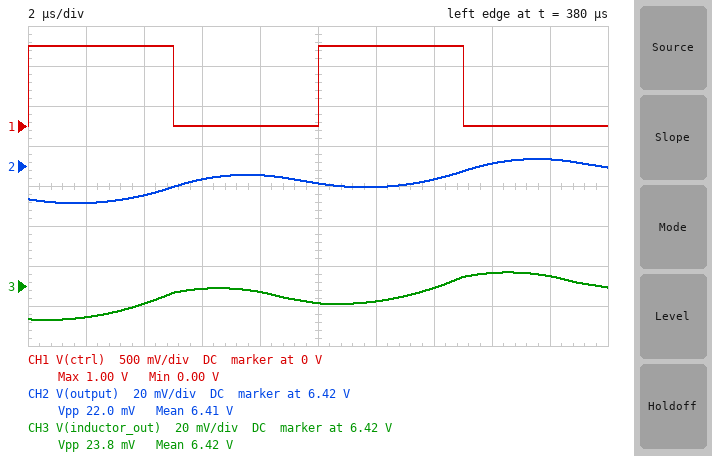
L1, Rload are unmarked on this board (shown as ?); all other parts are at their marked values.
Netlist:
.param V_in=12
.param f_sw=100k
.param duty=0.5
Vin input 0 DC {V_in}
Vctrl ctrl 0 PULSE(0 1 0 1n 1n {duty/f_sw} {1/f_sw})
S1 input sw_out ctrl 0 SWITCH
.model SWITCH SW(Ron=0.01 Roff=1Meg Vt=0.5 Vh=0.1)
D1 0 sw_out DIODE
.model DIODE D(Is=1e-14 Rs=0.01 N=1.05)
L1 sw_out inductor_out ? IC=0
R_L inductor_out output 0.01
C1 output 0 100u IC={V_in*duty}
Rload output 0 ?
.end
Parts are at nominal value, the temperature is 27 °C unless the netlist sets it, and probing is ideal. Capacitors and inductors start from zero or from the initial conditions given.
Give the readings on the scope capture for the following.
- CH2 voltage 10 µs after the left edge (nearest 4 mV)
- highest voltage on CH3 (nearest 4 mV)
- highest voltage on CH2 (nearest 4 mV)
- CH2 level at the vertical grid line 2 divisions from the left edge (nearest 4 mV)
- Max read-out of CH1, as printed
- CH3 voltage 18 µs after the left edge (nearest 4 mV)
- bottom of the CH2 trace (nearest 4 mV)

6.412 V
6.428 V
6.424 V
6.404 V
1.00 V
6.424 V
6.400 V
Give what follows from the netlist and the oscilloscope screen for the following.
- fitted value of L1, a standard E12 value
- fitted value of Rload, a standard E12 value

39 µH
27 Ω
